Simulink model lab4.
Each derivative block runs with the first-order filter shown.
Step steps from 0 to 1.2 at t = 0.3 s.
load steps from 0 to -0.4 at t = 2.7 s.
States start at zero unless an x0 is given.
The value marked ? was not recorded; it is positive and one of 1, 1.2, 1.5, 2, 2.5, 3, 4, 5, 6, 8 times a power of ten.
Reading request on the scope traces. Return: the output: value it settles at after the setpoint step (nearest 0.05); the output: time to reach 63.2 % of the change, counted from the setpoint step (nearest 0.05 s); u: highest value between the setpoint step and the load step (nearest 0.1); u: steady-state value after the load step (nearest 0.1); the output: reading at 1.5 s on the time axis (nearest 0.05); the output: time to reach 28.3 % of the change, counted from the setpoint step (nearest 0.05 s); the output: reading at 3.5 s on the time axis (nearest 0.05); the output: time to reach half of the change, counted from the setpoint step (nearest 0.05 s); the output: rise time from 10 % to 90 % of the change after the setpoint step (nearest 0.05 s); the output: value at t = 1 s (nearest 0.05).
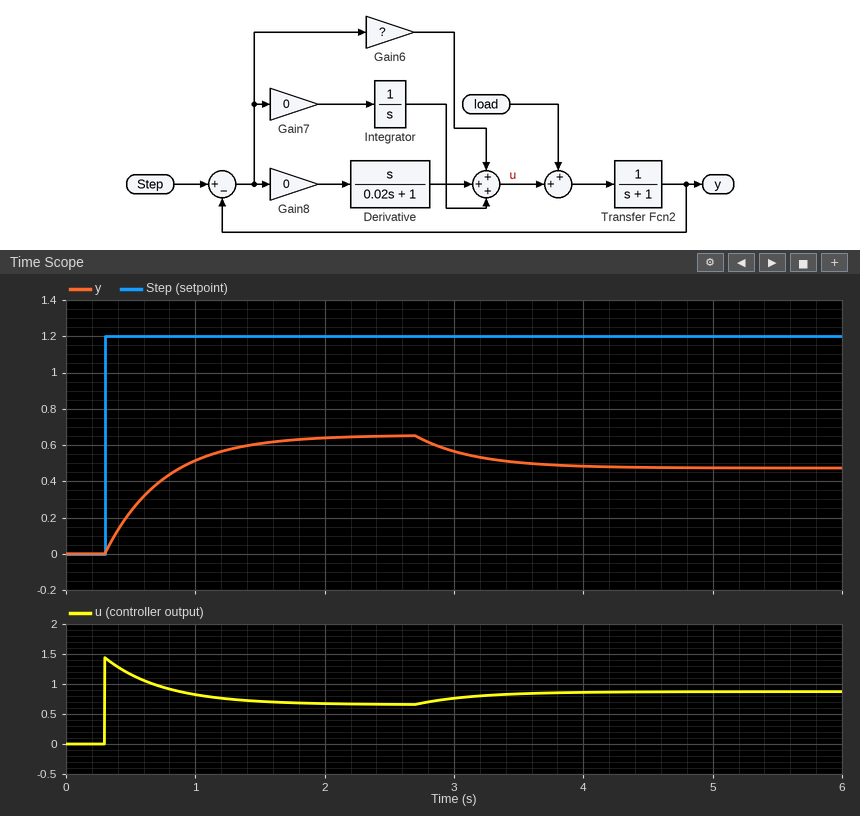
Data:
0.65
0.45 s
1.4
0.9
0.60
0.15 s
0.50
0.30 s
1.00 s
0.50
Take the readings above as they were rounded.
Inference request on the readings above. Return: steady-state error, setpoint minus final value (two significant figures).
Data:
0.55
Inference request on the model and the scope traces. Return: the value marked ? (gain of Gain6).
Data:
1.2
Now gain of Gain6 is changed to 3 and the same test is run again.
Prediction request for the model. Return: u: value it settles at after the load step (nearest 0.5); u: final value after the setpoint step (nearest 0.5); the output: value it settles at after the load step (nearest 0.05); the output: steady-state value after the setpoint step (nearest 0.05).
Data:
1.0
1.0
0.80
0.90
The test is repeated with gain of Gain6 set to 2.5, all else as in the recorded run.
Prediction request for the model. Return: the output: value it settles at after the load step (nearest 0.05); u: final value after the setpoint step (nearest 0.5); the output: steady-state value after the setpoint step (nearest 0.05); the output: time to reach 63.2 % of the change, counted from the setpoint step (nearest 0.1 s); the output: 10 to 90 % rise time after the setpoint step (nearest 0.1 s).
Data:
0.75
1.0
0.85
0.3 s
0.6 s
